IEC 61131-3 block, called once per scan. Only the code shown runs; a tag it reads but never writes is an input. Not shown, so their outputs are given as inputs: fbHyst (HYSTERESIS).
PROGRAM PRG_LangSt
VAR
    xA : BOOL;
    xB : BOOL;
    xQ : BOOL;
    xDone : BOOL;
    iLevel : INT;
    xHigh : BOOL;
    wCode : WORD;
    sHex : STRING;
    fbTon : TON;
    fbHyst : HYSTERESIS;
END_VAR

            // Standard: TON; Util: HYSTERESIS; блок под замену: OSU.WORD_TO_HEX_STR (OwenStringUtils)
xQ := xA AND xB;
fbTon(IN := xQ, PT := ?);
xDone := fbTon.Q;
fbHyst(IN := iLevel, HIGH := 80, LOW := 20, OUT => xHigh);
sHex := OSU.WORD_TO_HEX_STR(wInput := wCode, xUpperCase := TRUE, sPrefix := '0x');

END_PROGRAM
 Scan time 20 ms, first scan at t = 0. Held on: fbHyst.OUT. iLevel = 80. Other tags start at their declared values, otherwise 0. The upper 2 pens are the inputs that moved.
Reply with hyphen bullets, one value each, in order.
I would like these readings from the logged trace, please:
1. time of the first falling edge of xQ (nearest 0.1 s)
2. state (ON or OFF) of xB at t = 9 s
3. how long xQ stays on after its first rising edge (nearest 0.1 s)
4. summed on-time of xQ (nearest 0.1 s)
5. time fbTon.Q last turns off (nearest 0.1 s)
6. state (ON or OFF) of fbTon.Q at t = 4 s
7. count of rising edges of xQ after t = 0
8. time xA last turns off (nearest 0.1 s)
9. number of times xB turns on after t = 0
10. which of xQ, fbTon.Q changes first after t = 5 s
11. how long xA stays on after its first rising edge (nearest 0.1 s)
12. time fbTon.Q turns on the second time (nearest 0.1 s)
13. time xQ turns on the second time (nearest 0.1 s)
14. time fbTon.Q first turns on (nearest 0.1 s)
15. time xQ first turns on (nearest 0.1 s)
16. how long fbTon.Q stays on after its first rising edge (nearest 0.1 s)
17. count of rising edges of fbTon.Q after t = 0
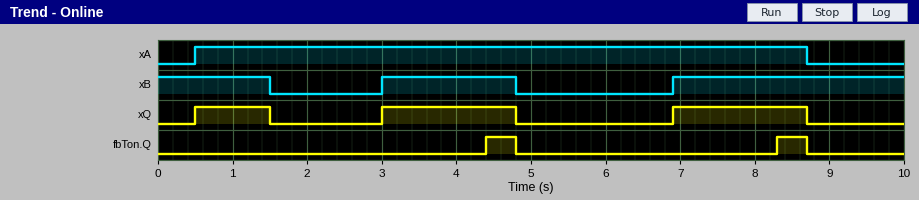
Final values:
- 1.5 s
- ON
- 1.0 s
- 4.6 s
- 8.7 s
- OFF
- 3
- 8.7 s
- 2
- xQ
- 8.2 s
- 8.3 s
- 3.0 s
- 4.4 s
- 0.5 s
- 0.4 s
- 2
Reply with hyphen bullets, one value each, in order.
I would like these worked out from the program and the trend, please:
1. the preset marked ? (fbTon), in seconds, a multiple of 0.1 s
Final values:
- 1.4 s
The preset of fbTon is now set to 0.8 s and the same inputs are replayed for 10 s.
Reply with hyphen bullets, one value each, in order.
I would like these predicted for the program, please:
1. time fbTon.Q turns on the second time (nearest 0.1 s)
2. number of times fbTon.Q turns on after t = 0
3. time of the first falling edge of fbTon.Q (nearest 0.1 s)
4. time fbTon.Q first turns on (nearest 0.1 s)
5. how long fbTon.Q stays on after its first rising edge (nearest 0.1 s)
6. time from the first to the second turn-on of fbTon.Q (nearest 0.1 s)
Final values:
- 3.8 s
- 3
- 1.5 s
- 1.3 s
- 0.2 s
- 2.5 s
